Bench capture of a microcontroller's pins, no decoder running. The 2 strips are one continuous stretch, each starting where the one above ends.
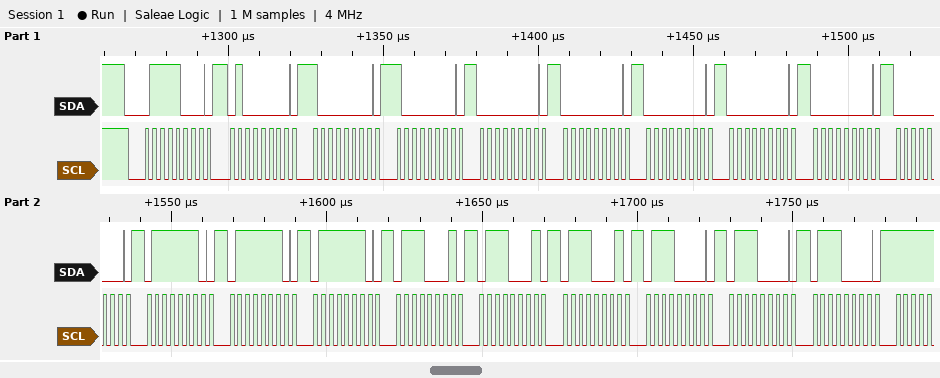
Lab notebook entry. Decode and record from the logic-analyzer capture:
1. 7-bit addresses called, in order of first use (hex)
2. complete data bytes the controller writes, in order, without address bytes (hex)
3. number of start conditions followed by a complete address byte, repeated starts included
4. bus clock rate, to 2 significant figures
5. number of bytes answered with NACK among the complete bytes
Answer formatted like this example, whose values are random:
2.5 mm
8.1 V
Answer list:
0x3C
40 80 80 00 00 00 00 00 00 7E 7E 7E 71 71 71 70 70 70
1
400 kHz
0
